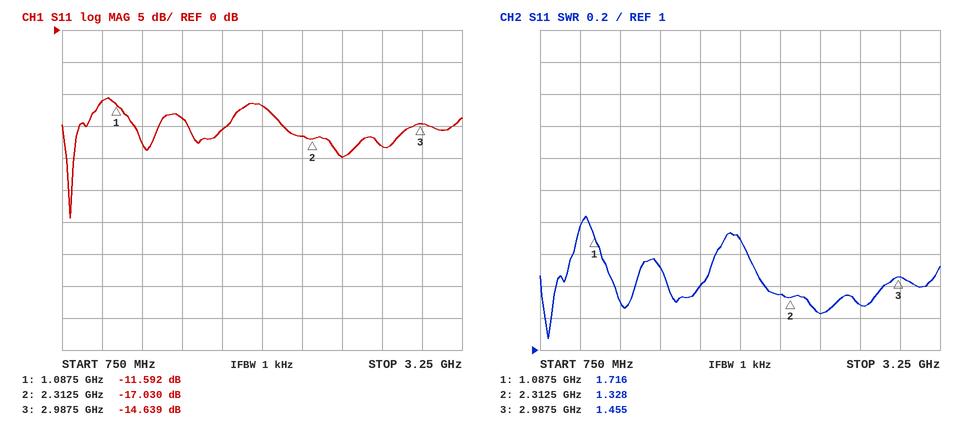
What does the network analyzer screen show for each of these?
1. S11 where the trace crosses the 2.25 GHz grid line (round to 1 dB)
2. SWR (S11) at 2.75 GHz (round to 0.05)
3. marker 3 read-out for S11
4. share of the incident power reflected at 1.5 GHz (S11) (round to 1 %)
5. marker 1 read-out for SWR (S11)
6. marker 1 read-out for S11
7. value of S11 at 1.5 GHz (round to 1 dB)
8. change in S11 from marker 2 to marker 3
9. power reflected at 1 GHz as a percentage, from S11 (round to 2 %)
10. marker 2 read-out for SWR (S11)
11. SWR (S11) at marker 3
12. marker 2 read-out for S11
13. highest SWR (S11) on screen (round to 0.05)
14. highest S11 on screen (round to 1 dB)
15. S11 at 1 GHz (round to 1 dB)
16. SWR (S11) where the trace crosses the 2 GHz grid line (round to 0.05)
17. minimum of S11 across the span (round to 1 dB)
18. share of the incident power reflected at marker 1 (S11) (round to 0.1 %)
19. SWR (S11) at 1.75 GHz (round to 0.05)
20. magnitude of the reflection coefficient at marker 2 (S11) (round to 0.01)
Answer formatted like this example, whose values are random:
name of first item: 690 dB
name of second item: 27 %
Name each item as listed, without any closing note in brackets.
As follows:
S11 where the trace crosses the 2.25 GHz grid line: -17 dB
SWR (S11) at 2.75 GHz: 1.30
marker 3 read-out for S11: -14.639 dB
share of the incident power reflected at 1.5 GHz (S11): 4 %
marker 1 read-out for SWR: 1.716
marker 1 read-out for S11: -11.592 dB
value of S11 at 1.5 GHz: -14 dB
change in S11 from marker 2 to marker 3: 2.391 dB
power reflected at 1 GHz as a percentage, from S11: 8 %
marker 2 read-out for SWR: 1.328
SWR (S11) at marker 3: 1.455
marker 2 read-out for S11: -17.030 dB
highest SWR (S11) on screen: 1.85
highest S11 on screen: -11 dB
S11 at 1 GHz: -11 dB
SWR (S11) where the trace crosses the 2 GHz grid line: 1.70
minimum of S11 across the span: -29 dB
share of the incident power reflected at marker 1 (S11): 6.9 %
SWR (S11) at 1.75 GHz: 1.40
magnitude of the reflection coefficient at marker 2 (S11): 0.14
